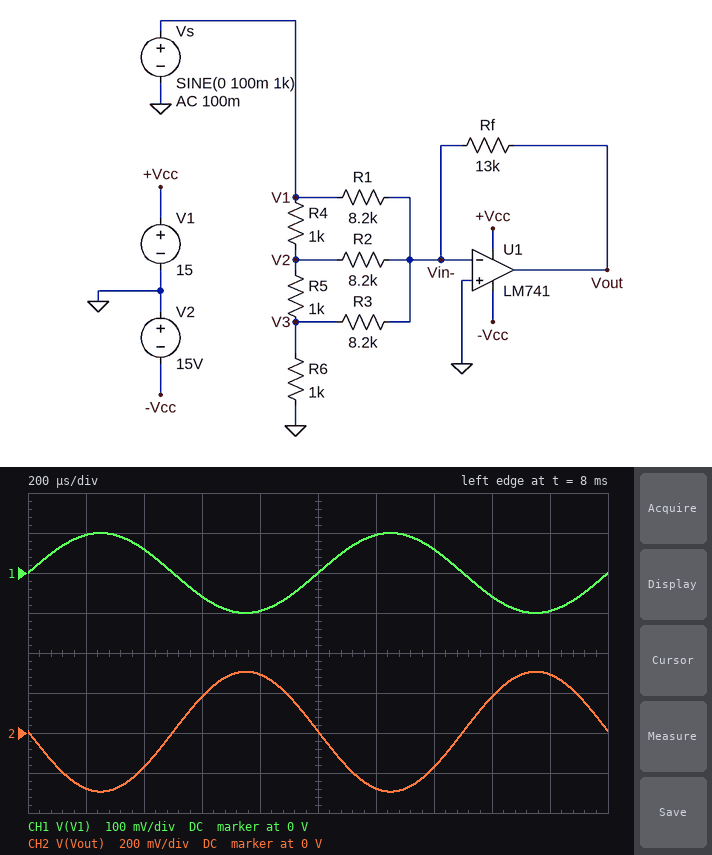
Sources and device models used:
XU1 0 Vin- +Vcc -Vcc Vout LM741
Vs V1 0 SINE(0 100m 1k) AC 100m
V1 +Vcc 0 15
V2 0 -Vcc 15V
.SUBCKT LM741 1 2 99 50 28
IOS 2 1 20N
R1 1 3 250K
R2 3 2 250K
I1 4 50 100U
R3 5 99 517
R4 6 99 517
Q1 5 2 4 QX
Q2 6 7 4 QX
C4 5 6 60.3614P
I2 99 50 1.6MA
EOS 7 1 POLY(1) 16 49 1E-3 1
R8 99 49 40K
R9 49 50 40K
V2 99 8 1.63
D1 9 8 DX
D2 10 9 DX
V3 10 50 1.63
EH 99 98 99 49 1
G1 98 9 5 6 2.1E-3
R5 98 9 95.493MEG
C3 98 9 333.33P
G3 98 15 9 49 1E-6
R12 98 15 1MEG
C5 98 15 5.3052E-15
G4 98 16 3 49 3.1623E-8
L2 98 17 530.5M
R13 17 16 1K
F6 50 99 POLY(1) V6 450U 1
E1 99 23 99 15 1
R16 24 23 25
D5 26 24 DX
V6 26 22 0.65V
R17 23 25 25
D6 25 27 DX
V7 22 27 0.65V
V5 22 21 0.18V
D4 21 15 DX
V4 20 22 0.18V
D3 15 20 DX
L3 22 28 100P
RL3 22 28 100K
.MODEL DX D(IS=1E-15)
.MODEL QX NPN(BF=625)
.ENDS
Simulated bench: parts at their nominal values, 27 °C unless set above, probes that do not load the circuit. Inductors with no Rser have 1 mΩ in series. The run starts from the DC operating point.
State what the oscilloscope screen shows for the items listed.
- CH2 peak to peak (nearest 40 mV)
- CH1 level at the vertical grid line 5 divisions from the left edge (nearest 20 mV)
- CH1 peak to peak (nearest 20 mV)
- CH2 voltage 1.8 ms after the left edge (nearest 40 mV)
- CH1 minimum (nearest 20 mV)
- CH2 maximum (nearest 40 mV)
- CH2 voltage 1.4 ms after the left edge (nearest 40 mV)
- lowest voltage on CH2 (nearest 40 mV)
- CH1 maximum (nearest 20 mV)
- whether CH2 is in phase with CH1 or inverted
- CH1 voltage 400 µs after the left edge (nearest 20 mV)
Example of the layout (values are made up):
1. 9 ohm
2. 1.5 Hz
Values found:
1. 600 mV
2. 0 V
3. 200 mV
4. 280 mV
5. -100 mV
6. 320 mV
7. -160 mV
8. -280 mV
9. 100 mV
10. inverted
11. 60 mV
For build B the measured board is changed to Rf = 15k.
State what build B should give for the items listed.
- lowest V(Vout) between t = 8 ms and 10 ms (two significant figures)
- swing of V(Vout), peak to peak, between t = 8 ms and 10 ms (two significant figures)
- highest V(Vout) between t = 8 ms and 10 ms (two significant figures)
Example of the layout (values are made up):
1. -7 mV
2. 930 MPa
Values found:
1. -340 mV
2. 690 mV
3. 350 mV
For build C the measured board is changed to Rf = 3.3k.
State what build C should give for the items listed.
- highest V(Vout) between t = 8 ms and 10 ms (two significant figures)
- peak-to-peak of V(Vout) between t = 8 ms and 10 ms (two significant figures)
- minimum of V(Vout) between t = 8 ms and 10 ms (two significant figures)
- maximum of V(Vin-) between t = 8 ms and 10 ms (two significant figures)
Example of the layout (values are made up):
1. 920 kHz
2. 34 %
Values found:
1. 79 mV
2. 150 mV
3. -74 mV
4. 1.1 mV
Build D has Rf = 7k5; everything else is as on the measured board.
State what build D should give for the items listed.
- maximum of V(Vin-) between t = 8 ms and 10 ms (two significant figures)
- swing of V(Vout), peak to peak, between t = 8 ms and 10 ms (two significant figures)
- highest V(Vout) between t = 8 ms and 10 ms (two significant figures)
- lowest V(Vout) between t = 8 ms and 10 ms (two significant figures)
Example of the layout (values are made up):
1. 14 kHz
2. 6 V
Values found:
1. 1.2 mV
2. 350 mV
3. 180 mV
4. -170 mV
